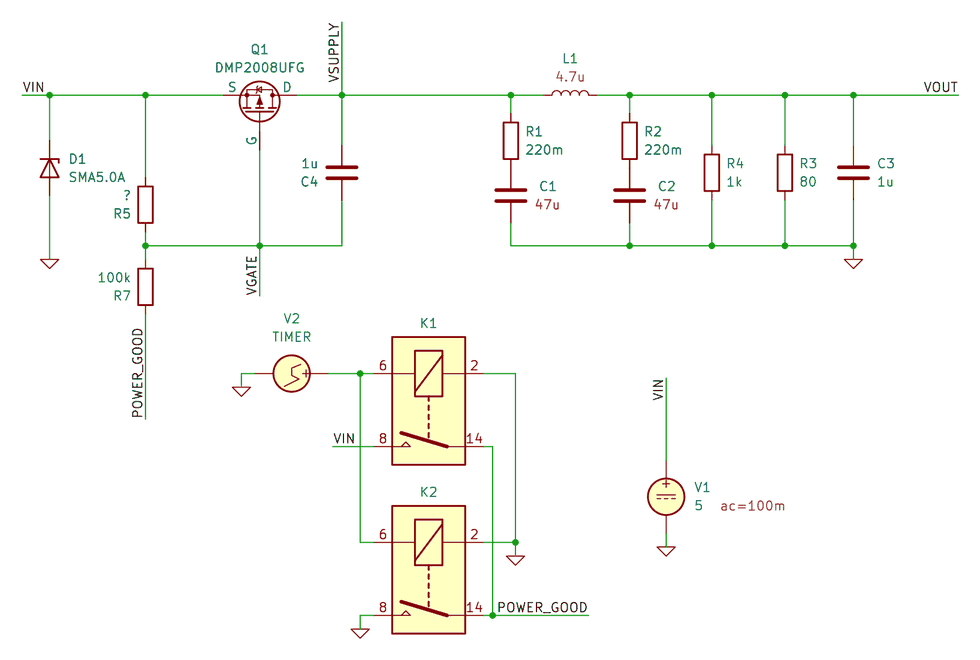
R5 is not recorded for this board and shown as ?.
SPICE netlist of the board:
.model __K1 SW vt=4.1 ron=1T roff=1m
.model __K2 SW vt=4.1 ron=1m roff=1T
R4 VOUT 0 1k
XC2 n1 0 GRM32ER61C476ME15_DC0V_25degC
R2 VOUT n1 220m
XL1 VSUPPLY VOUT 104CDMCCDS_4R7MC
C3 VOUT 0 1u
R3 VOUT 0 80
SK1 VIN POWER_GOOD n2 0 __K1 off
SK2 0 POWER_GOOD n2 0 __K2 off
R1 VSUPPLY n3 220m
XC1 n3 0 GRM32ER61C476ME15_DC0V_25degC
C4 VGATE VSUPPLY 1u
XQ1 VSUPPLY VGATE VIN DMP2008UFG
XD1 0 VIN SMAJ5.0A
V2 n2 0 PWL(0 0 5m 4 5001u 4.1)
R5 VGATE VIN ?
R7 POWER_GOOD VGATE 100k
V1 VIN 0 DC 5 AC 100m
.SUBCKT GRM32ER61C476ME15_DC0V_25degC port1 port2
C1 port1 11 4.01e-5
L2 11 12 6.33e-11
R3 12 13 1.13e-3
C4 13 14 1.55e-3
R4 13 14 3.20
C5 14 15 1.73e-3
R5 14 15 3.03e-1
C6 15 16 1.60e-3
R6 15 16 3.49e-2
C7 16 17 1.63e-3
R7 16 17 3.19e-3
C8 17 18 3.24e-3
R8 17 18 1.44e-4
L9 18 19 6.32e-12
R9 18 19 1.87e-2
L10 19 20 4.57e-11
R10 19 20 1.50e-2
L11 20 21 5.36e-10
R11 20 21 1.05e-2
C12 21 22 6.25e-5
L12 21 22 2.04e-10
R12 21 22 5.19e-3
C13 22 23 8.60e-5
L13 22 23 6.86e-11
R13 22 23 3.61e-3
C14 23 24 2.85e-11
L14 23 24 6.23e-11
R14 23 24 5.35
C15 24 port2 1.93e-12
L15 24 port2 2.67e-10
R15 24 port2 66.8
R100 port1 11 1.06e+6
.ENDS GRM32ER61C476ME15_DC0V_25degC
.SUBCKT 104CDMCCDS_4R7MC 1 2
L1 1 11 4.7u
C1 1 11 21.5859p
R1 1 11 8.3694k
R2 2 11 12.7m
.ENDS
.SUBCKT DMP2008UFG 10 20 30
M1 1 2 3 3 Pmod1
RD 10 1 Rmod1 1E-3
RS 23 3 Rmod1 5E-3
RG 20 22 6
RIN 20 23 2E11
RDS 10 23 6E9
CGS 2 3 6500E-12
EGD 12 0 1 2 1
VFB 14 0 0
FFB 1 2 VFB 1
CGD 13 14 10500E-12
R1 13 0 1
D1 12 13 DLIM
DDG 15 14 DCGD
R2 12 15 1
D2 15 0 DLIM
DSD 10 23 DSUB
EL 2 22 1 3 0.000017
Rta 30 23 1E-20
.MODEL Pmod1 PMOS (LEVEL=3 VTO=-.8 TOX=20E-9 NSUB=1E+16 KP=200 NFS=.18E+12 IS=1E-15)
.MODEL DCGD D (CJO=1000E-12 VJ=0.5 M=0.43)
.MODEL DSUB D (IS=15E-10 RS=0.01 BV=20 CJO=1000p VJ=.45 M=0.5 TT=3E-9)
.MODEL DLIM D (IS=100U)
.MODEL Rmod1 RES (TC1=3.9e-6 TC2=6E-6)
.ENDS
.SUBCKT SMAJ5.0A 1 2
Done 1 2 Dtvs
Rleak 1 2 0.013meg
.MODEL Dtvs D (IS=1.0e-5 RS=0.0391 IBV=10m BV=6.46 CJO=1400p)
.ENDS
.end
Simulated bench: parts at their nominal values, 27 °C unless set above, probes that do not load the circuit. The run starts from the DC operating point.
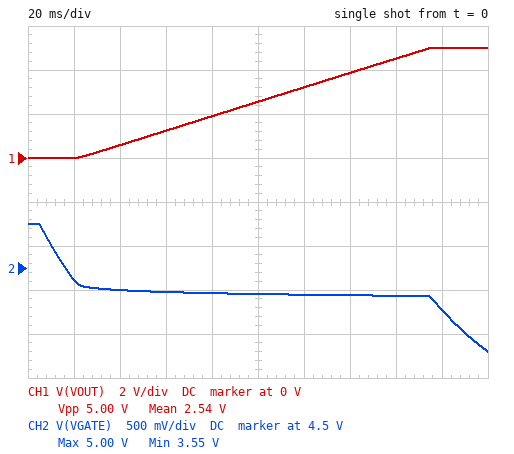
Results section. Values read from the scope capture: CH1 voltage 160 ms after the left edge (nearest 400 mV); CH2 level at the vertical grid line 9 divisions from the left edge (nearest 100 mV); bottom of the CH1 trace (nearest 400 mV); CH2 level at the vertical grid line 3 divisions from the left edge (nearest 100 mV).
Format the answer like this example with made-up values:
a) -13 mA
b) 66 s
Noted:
a) 4.4 V
b) 4.0 V
c) 0 V
d) 4.2 V
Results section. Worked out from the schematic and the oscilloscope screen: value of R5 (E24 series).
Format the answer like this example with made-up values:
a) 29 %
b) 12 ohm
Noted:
a) 91 kΩ
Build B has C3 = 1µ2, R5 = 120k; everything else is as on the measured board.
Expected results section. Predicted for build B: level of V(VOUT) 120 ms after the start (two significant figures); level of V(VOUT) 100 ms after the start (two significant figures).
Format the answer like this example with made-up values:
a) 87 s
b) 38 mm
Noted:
a) 3.4 V
b) 2.7 V
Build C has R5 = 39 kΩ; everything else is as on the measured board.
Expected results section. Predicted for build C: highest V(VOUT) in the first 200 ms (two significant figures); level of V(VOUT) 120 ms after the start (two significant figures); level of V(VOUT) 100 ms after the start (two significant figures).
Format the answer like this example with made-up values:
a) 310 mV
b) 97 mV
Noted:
a) 3.8 V
b) 2.1 V
c) 1.7 V
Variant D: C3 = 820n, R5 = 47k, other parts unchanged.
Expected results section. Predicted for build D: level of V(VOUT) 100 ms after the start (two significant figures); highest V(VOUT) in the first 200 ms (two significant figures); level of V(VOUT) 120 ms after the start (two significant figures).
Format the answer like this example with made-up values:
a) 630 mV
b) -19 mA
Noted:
a) 1.9 V
b) 4.4 V
c) 2.4 V
